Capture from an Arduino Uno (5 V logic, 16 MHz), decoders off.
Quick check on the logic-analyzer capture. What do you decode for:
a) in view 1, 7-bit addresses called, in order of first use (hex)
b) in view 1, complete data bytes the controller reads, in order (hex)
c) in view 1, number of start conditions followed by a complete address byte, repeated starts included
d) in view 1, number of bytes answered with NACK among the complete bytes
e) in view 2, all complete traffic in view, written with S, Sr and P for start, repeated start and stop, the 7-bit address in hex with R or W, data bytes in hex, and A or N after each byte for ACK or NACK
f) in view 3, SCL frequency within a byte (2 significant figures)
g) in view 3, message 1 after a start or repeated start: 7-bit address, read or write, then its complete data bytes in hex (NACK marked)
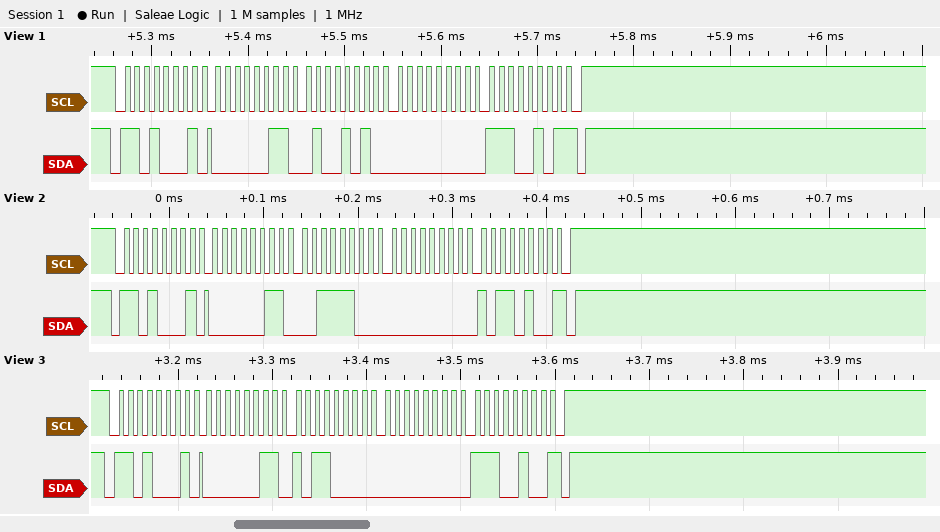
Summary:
0x68
03 4A 00 E5
1
1
S 68R A 03 A 3C A 00 A B4 N P
100 kHz
0x68 read: 03 B0 00 E4 NACK
